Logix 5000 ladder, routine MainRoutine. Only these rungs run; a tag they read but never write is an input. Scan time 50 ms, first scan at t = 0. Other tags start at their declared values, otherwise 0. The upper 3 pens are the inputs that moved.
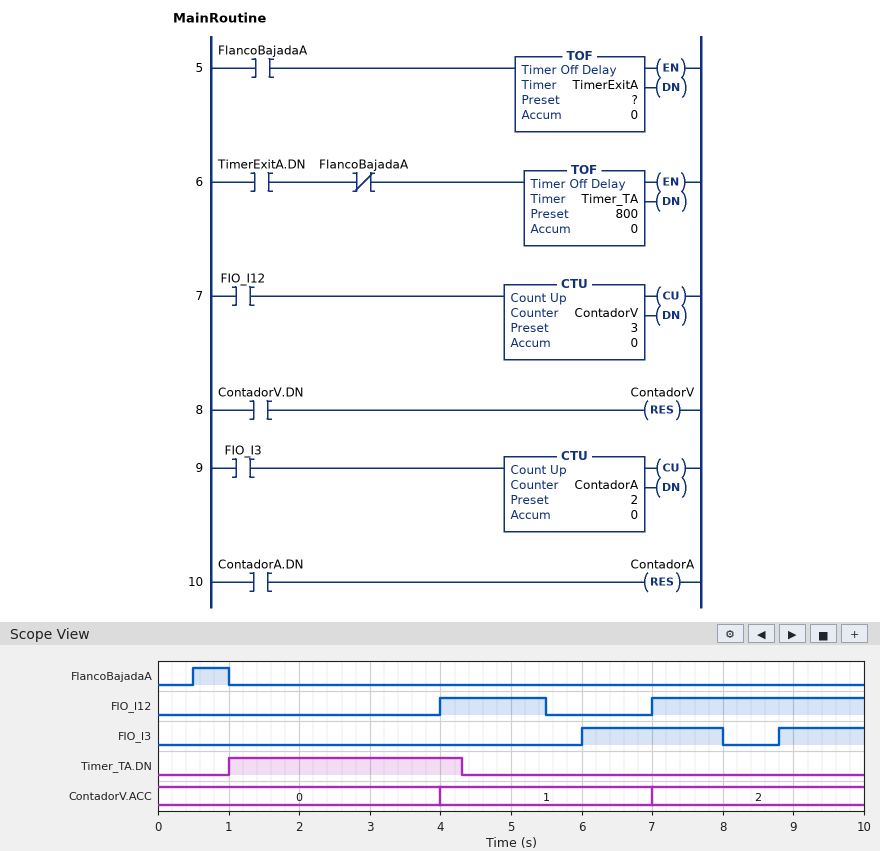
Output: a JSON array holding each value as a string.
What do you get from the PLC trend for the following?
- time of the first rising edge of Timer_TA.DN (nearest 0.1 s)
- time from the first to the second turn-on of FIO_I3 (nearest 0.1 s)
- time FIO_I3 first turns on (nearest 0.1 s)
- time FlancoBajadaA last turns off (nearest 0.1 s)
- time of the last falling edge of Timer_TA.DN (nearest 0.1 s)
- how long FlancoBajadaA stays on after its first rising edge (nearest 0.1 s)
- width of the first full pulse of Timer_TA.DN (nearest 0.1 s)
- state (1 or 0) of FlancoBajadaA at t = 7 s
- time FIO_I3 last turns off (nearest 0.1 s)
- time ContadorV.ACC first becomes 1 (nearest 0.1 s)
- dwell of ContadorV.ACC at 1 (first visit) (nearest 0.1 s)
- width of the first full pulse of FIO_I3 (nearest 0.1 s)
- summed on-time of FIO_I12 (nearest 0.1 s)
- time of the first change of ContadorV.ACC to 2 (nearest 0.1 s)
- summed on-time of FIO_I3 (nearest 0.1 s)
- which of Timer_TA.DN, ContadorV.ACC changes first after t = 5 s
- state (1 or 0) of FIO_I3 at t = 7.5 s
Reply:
["1.0 s", "2.8 s", "6.0 s", "1.0 s", "4.3 s", "0.5 s", "3.3 s", "0", "8.0 s", "4.0 s", "3.0 s", "2.0 s", "4.5 s", "7.0 s", "3.2 s", "ContadorV.ACC", "1"]
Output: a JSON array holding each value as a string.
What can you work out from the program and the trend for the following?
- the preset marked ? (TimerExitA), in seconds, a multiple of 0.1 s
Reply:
["2.5 s"]
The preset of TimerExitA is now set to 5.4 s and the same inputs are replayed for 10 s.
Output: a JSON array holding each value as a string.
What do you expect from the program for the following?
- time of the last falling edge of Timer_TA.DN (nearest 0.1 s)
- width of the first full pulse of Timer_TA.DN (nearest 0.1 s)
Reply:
["7.2 s", "6.2 s"]
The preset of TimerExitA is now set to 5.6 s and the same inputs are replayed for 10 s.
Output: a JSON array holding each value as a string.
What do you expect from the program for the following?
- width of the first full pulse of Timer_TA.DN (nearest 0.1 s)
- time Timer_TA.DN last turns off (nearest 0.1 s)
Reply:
["6.4 s", "7.4 s"]
